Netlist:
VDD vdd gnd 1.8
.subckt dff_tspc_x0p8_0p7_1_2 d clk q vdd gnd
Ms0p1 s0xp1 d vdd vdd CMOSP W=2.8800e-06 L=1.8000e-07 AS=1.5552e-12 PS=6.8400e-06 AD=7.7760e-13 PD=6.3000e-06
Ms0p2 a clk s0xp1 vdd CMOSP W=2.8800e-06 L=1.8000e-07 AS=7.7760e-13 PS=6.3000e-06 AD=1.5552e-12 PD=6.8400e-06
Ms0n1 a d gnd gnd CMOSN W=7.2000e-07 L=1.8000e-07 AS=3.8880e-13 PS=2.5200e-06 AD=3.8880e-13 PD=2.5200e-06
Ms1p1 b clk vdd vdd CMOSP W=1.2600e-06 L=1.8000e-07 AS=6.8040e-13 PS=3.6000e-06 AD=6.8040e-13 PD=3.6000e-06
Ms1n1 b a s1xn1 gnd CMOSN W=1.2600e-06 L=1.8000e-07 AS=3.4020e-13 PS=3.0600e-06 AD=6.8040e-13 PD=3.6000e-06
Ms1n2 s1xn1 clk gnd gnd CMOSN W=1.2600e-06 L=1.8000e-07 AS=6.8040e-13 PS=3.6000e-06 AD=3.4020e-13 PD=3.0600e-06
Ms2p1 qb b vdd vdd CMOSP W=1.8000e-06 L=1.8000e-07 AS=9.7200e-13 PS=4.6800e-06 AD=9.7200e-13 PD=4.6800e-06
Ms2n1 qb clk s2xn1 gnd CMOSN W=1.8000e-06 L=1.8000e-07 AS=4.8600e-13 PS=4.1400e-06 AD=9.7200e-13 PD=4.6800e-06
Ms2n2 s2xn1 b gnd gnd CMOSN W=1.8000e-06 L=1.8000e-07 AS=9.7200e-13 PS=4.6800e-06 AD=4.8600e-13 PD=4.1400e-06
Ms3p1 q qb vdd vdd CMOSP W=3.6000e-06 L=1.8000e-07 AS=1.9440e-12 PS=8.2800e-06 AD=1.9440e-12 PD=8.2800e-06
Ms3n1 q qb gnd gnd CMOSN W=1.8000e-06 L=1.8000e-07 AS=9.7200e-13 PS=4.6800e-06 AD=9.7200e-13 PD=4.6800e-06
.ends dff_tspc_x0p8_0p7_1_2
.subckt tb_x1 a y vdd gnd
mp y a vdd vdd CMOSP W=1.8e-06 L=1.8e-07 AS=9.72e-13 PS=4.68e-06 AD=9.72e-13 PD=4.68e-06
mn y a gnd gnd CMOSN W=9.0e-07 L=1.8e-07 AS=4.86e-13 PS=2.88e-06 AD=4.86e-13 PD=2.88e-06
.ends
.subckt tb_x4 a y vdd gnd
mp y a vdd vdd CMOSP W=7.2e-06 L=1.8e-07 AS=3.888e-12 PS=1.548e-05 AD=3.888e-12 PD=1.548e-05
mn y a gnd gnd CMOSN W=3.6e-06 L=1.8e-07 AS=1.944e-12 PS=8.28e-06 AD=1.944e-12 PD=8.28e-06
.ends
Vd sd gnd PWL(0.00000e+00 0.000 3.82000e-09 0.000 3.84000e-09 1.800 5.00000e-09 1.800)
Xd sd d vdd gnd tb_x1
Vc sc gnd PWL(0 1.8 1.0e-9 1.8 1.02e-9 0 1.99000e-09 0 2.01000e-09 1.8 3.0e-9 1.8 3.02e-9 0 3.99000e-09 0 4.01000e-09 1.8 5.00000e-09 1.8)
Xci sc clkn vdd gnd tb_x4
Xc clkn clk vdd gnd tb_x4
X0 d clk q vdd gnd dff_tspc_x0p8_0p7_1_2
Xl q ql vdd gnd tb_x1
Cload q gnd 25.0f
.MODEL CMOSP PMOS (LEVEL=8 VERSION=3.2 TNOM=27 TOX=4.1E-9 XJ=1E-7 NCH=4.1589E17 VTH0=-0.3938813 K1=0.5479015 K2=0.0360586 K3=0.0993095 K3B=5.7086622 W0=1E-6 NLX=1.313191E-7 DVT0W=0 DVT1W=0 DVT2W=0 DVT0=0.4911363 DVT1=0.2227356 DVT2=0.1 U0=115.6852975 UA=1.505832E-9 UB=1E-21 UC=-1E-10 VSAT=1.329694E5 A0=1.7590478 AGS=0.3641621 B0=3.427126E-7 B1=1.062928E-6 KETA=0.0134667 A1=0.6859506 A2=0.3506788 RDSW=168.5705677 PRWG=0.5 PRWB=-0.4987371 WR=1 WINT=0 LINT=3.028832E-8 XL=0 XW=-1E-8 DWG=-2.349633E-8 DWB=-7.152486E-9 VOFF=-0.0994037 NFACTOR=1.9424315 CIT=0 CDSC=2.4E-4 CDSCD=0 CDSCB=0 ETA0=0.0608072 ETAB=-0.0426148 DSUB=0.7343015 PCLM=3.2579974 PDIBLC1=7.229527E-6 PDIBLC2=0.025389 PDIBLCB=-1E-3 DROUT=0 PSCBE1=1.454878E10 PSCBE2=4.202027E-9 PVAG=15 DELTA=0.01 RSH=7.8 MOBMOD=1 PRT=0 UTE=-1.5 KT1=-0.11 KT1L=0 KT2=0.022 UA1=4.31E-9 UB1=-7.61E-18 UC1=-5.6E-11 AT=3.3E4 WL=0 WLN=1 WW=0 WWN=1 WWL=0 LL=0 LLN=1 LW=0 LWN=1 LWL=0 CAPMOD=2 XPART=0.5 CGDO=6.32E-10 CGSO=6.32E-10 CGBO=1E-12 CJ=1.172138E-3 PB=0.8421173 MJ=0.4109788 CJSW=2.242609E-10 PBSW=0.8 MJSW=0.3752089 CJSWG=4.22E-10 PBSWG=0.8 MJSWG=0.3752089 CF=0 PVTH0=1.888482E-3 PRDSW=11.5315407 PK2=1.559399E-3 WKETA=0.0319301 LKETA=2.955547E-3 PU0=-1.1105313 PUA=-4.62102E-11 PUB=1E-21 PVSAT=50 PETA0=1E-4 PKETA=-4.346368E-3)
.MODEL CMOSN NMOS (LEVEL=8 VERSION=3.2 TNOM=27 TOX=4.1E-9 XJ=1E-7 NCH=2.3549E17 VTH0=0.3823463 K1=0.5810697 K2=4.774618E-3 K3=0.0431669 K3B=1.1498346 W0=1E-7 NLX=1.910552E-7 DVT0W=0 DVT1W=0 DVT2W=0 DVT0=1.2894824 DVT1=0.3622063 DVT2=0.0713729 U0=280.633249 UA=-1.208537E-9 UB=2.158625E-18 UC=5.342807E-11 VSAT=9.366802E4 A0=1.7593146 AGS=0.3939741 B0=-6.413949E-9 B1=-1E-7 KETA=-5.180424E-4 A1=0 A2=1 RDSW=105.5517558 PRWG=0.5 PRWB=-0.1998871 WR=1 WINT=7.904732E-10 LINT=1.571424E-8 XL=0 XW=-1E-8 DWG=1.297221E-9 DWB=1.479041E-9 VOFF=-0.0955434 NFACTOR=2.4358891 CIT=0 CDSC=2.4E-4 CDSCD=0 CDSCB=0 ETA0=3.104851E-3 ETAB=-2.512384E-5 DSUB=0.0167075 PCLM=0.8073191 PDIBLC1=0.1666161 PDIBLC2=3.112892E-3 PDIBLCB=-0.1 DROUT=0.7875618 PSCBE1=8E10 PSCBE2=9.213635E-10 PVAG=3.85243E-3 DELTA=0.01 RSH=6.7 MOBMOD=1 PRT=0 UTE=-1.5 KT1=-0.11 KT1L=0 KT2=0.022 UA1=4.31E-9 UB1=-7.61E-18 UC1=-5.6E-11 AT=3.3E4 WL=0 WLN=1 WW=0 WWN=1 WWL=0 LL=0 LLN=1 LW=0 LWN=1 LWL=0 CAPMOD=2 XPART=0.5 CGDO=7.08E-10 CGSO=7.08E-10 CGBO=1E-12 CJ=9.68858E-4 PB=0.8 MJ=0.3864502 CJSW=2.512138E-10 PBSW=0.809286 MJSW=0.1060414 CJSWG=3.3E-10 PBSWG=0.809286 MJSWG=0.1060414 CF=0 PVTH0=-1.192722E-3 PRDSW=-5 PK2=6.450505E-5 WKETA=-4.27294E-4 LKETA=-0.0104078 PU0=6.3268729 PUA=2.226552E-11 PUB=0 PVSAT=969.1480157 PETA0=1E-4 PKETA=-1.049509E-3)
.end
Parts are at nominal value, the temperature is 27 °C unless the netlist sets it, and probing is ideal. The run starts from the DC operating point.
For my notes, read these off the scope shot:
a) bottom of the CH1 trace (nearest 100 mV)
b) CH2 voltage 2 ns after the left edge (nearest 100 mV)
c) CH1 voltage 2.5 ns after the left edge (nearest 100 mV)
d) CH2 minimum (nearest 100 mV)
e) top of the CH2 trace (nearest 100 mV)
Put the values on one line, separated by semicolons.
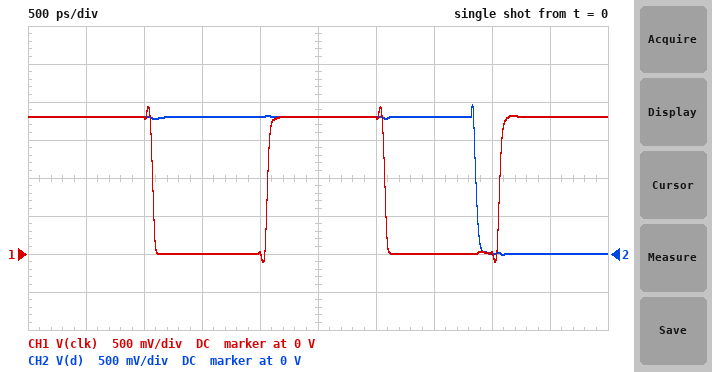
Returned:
-100 mV; 1.8 V; 1.8 V; 0 V; 2.0 V
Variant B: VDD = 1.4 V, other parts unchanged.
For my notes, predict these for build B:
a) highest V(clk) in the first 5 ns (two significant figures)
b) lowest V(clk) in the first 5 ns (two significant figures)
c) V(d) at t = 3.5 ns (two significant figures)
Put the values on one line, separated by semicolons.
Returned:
1.5 V; -160 mV; 1.4 V
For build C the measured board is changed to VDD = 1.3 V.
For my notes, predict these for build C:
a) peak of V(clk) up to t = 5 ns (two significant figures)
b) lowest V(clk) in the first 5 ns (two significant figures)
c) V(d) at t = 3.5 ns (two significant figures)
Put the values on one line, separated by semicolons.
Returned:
1.4 V; -170 mV; 1.3 V
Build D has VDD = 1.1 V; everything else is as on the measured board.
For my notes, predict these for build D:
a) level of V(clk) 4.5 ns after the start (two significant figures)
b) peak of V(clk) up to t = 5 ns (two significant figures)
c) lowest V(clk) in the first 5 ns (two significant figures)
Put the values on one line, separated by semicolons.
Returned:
1.1 V; 1.2 V; -200 mV
